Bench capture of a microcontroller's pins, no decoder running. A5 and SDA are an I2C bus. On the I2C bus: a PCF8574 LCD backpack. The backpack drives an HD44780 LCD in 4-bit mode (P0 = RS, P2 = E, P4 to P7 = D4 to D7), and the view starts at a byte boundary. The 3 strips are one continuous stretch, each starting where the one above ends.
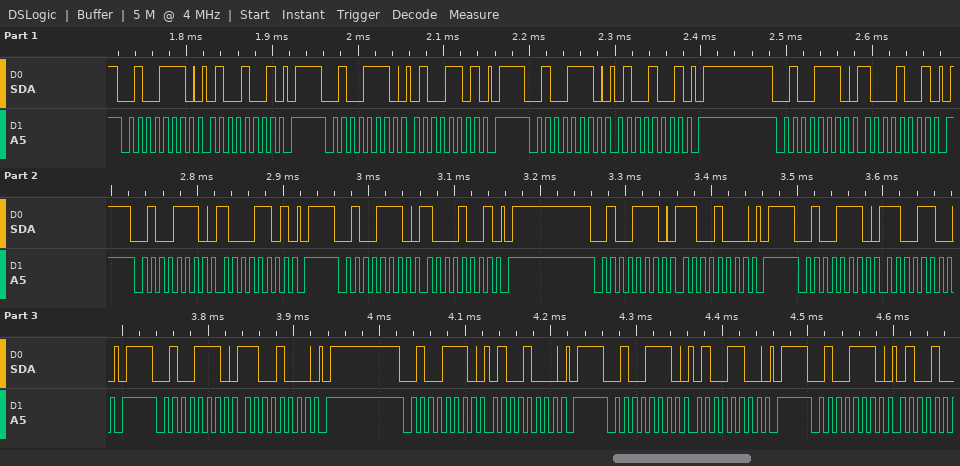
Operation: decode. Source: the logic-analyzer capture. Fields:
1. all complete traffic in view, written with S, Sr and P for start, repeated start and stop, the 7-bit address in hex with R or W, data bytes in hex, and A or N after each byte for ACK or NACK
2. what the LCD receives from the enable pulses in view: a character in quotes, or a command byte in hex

S 27W A 49 A P S 27W A 4D A P S 27W A 49 A P S 27W A 89 A P S 27W A 8D A P S 27W A 89 A P S 27W A C8 A P S 27W A CC A P S 27W A C8 A P S 27W A 48 A P S 27W A 4C A P S 27W A
'H'
